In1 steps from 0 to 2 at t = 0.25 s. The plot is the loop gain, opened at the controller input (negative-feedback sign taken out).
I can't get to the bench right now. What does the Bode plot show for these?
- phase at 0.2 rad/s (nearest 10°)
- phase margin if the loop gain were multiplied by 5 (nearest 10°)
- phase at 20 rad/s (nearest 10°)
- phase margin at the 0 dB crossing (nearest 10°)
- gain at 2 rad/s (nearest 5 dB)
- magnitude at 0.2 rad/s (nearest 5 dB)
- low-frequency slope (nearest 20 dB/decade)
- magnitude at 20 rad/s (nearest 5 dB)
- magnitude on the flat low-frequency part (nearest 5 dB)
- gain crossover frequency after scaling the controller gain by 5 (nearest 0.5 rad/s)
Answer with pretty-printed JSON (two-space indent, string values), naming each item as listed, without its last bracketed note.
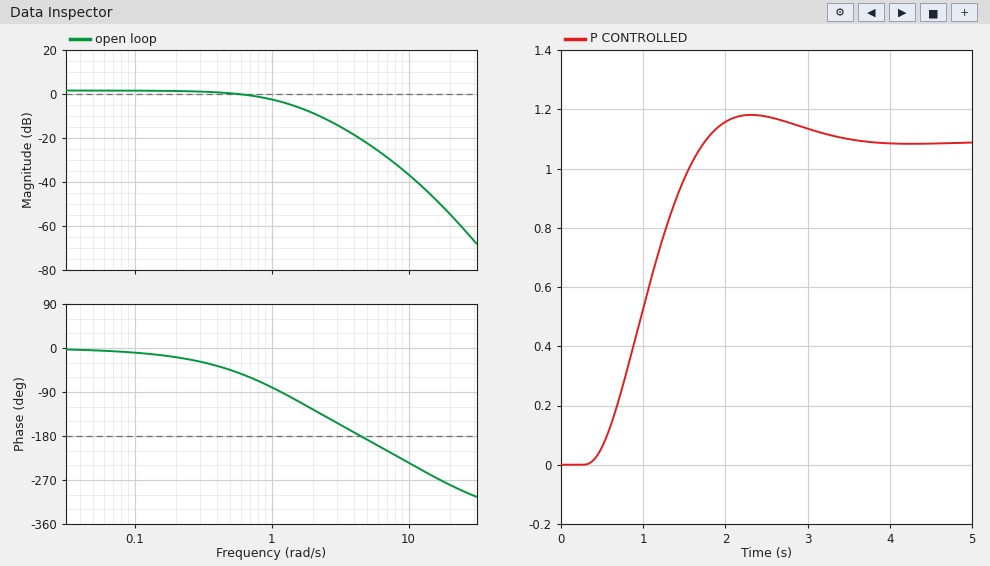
{
  "phase at 0.2 rad/s": "-20°",
  "phase margin if the loop gain were multiplied by 5": "30°",
  "phase at 20 rad/s": "-280°",
  "phase margin at the 0 dB crossing": "130°",
  "gain at 2 rad/s": "-10 dB",
  "magnitude at 0.2 rad/s": "0 dB",
  "low-frequency slope": "0 dB/decade",
  "magnitude at 20 rad/s": "-55 dB",
  "magnitude on the flat low-frequency part": "0 dB",
  "gain crossover frequency after scaling the controller gain by 5": "3.0 rad/s"
}
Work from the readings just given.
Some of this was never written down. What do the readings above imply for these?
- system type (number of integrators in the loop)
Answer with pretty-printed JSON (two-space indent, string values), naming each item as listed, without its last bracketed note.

{
  "system type": "0"
}
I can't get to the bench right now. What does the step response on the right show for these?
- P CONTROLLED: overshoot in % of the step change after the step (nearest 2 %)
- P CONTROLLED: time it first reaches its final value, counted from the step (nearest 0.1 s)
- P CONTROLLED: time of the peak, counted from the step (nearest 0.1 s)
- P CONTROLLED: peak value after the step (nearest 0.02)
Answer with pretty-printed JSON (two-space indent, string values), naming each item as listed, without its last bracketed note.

{
  "P CONTROLLED: overshoot in % of the step change after the step": "8 %",
  "P CONTROLLED: time it first reaches its final value, counted from the step": "1.5 s",
  "P CONTROLLED: time of the peak, counted from the step": "2.1 s",
  "P CONTROLLED: peak value after the step": "1.18"
}
